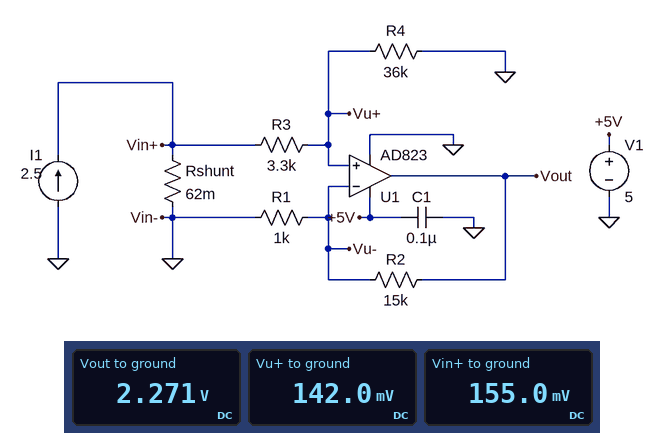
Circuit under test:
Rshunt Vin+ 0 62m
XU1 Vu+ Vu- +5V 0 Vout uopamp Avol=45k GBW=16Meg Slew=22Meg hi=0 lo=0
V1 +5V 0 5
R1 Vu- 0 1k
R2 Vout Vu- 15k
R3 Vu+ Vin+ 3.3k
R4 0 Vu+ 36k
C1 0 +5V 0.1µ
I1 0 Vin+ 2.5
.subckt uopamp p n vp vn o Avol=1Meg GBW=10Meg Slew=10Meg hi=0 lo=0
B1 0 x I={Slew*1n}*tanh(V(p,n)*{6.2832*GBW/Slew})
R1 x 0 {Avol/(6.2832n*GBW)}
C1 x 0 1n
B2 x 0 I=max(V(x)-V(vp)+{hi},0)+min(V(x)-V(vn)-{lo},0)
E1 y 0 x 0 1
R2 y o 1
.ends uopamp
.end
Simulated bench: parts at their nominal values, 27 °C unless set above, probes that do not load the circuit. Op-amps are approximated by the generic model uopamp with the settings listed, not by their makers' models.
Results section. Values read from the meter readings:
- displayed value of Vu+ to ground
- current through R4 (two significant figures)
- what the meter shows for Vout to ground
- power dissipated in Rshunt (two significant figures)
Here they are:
142.0 mV
3.9 µA
2.271 V
390 mW
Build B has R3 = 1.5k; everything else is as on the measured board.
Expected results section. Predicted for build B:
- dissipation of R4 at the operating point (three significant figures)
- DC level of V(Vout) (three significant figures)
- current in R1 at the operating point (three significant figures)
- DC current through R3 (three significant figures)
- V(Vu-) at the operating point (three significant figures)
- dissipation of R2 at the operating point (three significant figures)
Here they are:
615 nW
2.38 V
149 µA
4.13 µA
149 mV
332 µW
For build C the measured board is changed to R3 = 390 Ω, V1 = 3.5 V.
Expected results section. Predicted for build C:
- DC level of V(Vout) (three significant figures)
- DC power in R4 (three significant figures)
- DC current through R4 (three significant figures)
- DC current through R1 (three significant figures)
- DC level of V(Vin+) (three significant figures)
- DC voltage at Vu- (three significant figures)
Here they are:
2.45 V
653 nW
4.26 µA
153 µA
155 mV
153 mV
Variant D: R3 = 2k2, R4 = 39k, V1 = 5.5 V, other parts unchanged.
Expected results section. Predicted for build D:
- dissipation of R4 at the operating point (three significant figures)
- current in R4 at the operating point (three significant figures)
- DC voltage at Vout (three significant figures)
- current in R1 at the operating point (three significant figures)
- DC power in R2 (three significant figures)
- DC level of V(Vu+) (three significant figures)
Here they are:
552 nW
3.76 µA
2.35 V
147 µA
323 µW
147 mV
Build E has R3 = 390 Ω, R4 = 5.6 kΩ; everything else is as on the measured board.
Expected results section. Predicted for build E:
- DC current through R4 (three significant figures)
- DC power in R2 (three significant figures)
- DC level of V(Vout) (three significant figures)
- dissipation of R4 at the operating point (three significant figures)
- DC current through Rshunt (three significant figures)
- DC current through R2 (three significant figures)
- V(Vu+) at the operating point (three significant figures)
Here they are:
25.9 µA
315 µW
2.32 V
3.75 µW
2.50 A
145 µA
145 mV
